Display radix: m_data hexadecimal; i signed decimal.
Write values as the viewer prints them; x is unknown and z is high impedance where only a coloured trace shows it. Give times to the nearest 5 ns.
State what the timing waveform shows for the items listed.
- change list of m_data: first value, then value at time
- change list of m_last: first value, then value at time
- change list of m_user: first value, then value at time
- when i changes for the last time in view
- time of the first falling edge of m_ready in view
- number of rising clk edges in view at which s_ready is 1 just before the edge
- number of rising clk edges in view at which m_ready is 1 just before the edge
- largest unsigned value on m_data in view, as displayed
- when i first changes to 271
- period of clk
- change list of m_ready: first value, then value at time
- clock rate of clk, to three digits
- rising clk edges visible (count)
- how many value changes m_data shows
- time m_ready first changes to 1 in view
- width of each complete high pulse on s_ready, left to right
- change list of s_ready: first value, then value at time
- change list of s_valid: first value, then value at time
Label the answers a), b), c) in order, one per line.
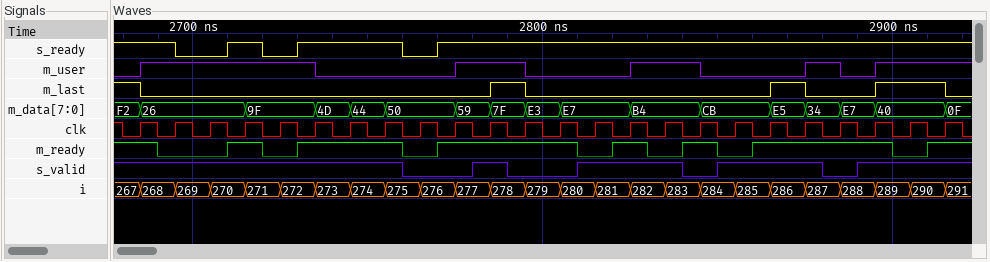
a) F2, 26 at 2685 ns, 9F at 2715 ns, 4D at 2735 ns, 44 at 2745 ns, 50 at 2755 ns, 59 at 2775 ns, 7F at 2785 ns, E3 at 2795 ns, E7 at 2805 ns, B4 at 2825 ns, CB at 2845 ns, E5 at 2865 ns, 34 at 2875 ns, E7 at 2885 ns, 40 at 2895 ns, 0F at 2915 ns
b) 1, 0 at 2685 ns, 1 at 2785 ns, 0 at 2795 ns, 1 at 2865 ns, 0 at 2875 ns, 1 at 2895 ns, 0 at 2915 ns
c) 0, 1 at 2685 ns, 0 at 2735 ns, 1 at 2775 ns, 0 at 2795 ns, 1 at 2825 ns, 0 at 2845 ns, 1 at 2875 ns, 0 at 2885 ns, 1 at 2895 ns
d) 2915 ns
e) 2690 ns
f) 21
g) 16
h) F2
i) 2715 ns
j) 10 ns
k) 1, 0 at 2690 ns, 1 at 2710 ns, 0 at 2720 ns, 1 at 2730 ns, 0 at 2760 ns, 1 at 2770 ns, 0 at 2810 ns, 1 at 2820 ns, 0 at 2830 ns, 1 at 2840 ns, 0 at 2850 ns, 1 at 2860 ns, 0 at 2900 ns, 1 at 2910 ns
l) 100 MHz
m) 24
n) 16
o) 2710 ns
p) 10 ns, 30 ns
q) 1, 0 at 2695 ns, 1 at 2710 ns, 0 at 2720 ns, 1 at 2730 ns, 0 at 2760 ns, 1 at 2770 ns
r) 1, 0 at 2760 ns, 1 at 2780 ns, 0 at 2790 ns, 1 at 2810 ns, 0 at 2840 ns, 1 at 2850 ns, 0 at 2880 ns, 1 at 2890 ns
